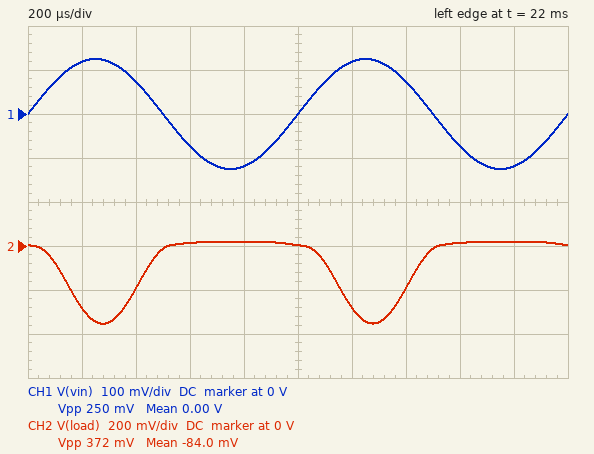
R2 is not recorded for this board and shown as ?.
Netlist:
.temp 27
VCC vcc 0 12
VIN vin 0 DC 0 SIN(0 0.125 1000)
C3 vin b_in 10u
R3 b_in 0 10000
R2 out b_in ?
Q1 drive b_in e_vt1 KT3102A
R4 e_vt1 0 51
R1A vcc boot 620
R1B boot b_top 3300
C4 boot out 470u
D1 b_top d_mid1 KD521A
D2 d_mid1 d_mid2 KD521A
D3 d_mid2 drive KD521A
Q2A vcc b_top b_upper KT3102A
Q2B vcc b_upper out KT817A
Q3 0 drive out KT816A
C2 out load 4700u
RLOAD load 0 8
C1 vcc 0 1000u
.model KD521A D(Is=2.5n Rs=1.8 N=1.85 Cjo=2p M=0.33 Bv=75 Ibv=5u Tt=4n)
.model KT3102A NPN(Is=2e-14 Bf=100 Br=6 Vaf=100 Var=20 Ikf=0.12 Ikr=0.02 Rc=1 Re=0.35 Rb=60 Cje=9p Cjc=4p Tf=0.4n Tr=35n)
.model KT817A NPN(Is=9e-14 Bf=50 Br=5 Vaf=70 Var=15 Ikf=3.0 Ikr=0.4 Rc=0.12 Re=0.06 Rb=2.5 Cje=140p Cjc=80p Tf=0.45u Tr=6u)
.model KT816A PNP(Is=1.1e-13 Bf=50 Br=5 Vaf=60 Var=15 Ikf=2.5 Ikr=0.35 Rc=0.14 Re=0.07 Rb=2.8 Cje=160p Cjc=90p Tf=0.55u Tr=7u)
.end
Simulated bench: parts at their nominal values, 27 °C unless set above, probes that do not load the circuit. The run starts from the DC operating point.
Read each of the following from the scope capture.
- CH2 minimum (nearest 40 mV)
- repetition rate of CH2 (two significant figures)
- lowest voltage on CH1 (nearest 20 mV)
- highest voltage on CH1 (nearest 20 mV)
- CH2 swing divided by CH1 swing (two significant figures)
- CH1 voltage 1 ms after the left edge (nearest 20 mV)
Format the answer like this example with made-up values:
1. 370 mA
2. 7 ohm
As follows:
1. -360 mV
2. 1.0 kHz
3. -120 mV
4. 120 mV
5. 1.5
6. 0 V
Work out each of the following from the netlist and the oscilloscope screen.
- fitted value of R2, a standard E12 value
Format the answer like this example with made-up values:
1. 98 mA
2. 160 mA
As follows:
1. 180 kΩ
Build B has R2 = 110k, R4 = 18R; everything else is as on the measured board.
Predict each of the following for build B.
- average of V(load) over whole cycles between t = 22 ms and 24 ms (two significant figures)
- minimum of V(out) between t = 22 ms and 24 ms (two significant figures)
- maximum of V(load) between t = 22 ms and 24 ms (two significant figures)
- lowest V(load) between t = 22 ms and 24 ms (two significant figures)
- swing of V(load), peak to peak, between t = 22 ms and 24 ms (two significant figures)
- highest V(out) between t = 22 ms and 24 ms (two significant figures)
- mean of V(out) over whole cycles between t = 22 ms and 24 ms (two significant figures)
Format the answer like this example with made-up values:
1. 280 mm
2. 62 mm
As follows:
1. 630 mV
2. 7.3 V
3. 2.4 V
4. -1.5 V
5. 3.9 V
6. 11 V
7. 9.4 V
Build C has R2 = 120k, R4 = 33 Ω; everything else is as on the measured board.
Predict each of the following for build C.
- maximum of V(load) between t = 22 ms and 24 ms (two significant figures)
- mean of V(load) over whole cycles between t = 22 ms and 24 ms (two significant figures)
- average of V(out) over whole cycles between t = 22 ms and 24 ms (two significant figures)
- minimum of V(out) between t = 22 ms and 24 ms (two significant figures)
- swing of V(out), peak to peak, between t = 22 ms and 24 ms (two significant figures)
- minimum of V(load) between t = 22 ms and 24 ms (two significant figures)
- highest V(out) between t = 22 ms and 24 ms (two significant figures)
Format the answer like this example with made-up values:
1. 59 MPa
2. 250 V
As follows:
1. 1.9 V
2. 540 mV
3. 9.8 V
4. 8.3 V
5. 2.9 V
6. -1.0 V
7. 11 V
